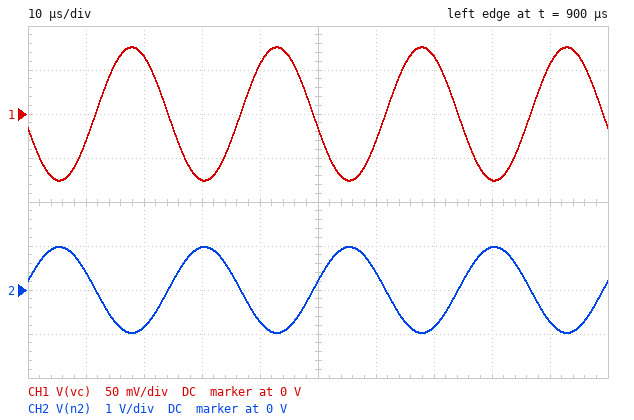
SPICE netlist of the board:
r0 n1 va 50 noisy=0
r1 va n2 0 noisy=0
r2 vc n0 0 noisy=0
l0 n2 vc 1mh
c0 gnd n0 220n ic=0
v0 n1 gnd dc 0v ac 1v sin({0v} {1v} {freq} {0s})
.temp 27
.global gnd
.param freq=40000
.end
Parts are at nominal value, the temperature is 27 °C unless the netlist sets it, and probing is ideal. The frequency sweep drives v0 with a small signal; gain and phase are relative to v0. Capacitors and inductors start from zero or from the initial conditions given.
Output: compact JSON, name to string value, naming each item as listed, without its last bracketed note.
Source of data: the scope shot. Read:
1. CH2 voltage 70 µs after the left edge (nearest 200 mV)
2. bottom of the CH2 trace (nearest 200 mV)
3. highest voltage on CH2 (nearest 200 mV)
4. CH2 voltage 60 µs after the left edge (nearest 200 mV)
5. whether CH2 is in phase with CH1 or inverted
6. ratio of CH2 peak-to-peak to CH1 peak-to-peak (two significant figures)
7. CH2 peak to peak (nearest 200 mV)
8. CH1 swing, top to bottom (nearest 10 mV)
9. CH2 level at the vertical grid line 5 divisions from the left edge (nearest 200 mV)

{"CH2 voltage 70 µs after the left edge": "-800 mV", "bottom of the CH2 trace": "-1.0 V", "highest voltage on CH2": "1.0 V", "CH2 voltage 60 µs after the left edge": "400 mV", "whether CH2 is in phase with CH1 or inverted": "inverted", "ratio of CH2 peak-to-peak to CH1 peak-to-peak": "13", "CH2 peak to peak": "2.0 V", "CH1 swing, top to bottom": "150 mV", "CH2 level at the vertical grid line 5 divisions from the left edge": "200 mV"}
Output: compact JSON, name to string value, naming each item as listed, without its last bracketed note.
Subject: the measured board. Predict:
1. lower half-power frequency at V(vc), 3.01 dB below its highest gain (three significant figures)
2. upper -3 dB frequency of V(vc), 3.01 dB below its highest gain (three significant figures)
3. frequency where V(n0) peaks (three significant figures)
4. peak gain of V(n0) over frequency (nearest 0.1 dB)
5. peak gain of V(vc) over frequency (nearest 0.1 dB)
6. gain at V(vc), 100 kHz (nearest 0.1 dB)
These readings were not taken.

{"lower half-power frequency at V(vc), 3.01 dB below its highest gain": "2.07 kHz", "upper -3 dB frequency of V(vc), 3.01 dB below its highest gain": "12.8 kHz", "frequency where V(n0) peaks": "9.14 kHz", "peak gain of V(n0) over frequency": "3.2 dB", "peak gain of V(vc) over frequency": "3.2 dB", "gain at V(vc), 100 kHz": "-38.7 dB"}
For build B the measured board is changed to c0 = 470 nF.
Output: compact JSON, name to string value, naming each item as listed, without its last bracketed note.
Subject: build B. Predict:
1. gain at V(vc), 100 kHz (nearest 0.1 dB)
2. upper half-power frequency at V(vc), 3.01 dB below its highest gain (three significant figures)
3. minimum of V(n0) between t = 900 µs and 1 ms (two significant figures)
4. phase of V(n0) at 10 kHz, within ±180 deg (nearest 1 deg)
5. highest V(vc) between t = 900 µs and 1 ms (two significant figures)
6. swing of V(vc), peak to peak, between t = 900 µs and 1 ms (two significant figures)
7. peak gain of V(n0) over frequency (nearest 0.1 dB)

{"gain at V(vc), 100 kHz": "-45.4 dB", "upper half-power frequency at V(vc), 3.01 dB below its highest gain": "8.45 kHz", "minimum of V(n0) between t = 900 µs and 1 ms": "-34 mV", "phase of V(n0) at 10 kHz, within ±180 deg": "-120 deg", "highest V(vc) between t = 900 µs and 1 ms": "34 mV", "swing of V(vc), peak to peak, between t = 900 µs and 1 ms": "68 mV", "peak gain of V(n0) over frequency": "0.8 dB"}
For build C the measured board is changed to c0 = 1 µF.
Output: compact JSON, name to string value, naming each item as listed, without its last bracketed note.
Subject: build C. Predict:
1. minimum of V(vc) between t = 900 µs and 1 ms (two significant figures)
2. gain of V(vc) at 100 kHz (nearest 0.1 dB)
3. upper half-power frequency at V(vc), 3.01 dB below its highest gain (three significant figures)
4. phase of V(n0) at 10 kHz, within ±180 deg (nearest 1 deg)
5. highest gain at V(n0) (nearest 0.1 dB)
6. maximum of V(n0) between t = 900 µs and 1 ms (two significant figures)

{"minimum of V(vc) between t = 900 µs and 1 ms": "-16 mV", "gain of V(vc) at 100 kHz": "-51.9 dB", "upper half-power frequency at V(vc), 3.01 dB below its highest gain": "4.45 kHz", "phase of V(n0) at 10 kHz, within ±180 deg": "-133 deg", "highest gain at V(n0)": "0 dB", "maximum of V(n0) between t = 900 µs and 1 ms": "16 mV"}
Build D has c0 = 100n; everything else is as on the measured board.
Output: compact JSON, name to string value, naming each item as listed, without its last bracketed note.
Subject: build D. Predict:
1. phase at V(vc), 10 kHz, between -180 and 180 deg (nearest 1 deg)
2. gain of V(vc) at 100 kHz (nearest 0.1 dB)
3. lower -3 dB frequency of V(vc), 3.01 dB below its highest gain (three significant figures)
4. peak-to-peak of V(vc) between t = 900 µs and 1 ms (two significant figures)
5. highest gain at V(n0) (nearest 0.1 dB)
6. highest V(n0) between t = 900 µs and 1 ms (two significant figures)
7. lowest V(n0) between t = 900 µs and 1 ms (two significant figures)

{"phase at V(vc), 10 kHz, between -180 and 180 deg": "-27 deg", "gain of V(vc) at 100 kHz": "-31.7 dB", "lower -3 dB frequency of V(vc), 3.01 dB below its highest gain": "9.96 kHz", "peak-to-peak of V(vc) between t = 900 µs and 1 ms": "370 mV", "highest gain at V(n0)": "6.3 dB", "highest V(n0) between t = 900 µs and 1 ms": "180 mV", "lowest V(n0) between t = 900 µs and 1 ms": "-180 mV"}
